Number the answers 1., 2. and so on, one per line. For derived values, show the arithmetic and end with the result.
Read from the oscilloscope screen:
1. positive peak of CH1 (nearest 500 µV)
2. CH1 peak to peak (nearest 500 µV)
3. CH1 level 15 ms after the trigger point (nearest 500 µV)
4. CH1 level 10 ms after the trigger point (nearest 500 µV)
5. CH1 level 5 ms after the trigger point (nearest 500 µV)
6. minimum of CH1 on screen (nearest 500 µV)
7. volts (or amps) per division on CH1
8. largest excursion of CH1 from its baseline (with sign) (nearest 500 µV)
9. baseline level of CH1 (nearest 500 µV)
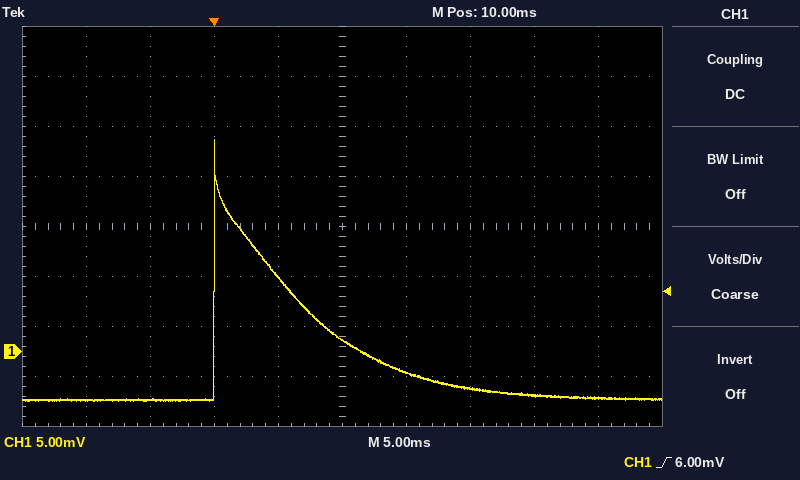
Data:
1. 21.0 mV
2. 21.0 mV − (-5.0 mV) = 26.0 mV
3. -2.0 mV
4. 1.0 mV
5. 7.5 mV
6. -5.0 mV
7. 5 mV
8. 21.0 mV − (-5.0 mV) = +26.0 mV
9. -5.0 mV
